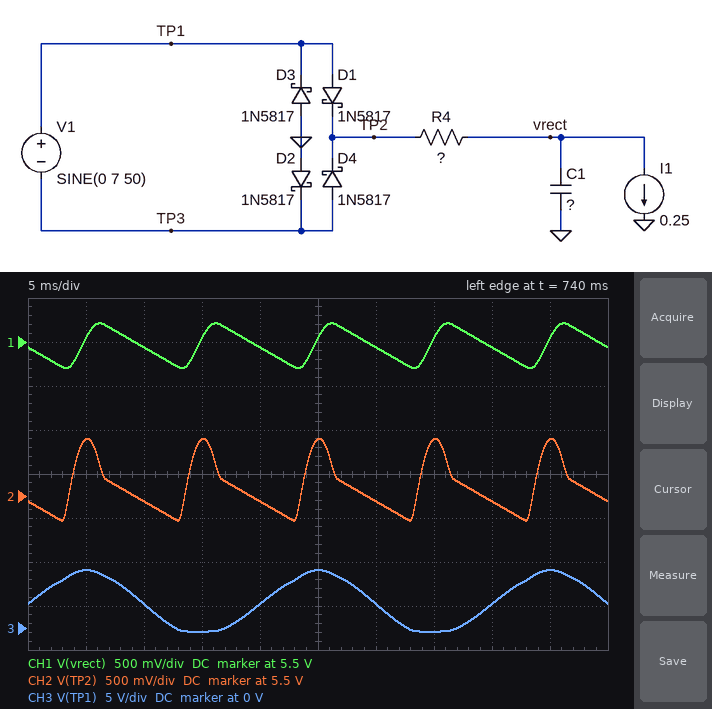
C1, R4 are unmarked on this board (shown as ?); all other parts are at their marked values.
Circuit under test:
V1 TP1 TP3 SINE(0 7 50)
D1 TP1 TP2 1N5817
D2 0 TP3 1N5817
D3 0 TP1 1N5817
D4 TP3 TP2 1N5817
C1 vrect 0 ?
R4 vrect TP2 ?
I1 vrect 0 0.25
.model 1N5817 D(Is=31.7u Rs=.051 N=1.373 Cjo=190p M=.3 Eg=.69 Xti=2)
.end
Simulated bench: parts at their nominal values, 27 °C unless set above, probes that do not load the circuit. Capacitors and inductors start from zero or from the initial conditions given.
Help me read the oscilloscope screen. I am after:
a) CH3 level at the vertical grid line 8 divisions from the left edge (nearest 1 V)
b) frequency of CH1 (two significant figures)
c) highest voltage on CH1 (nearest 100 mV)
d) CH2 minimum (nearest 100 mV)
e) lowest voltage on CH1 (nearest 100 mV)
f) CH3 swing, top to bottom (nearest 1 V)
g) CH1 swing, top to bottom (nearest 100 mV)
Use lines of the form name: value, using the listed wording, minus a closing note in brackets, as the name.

CH3 level at the vertical grid line 8 divisions from the left edge: 3 V
frequency of CH1: 100 Hz
highest voltage on CH1: 5.7 V
CH2 minimum: 5.2 V
lowest voltage on CH1: 5.2 V
CH3 swing, top to bottom: 7 V
CH1 swing, top to bottom: 500 mV
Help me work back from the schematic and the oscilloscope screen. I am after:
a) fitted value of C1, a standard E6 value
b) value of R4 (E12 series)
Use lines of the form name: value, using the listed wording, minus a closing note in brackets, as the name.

fitted value of C1, a standard E6 value: 3.3 mF
value of R4: 0.56 Ω
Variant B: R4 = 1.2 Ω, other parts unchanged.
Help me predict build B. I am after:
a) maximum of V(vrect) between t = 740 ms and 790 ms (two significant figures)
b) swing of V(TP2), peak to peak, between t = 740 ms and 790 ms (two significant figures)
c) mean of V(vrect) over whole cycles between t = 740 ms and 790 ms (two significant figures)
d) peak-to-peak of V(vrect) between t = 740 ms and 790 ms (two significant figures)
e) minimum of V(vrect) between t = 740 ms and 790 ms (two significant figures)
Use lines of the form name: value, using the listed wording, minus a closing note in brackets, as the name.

maximum of V(vrect) between t = 740 ms and 790 ms: 5.3 V
swing of V(TP2), peak to peak, between t = 740 ms and 790 ms: 1.4 V
mean of V(vrect) over whole cycles between t = 740 ms and 790 ms: 5.0 V
peak-to-peak of V(vrect) between t = 740 ms and 790 ms: 470 mV
minimum of V(vrect) between t = 740 ms and 790 ms: 4.8 V
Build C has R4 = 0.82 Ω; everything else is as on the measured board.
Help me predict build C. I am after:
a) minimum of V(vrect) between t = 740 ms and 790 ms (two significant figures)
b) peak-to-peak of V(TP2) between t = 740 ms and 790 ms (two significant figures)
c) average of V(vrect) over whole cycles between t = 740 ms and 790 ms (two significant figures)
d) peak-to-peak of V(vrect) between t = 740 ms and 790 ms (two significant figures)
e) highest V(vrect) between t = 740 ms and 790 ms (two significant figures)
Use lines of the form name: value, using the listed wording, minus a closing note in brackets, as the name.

minimum of V(vrect) between t = 740 ms and 790 ms: 5.0 V
peak-to-peak of V(TP2) between t = 740 ms and 790 ms: 1.1 V
average of V(vrect) over whole cycles between t = 740 ms and 790 ms: 5.3 V
peak-to-peak of V(vrect) between t = 740 ms and 790 ms: 490 mV
highest V(vrect) between t = 740 ms and 790 ms: 5.5 V
